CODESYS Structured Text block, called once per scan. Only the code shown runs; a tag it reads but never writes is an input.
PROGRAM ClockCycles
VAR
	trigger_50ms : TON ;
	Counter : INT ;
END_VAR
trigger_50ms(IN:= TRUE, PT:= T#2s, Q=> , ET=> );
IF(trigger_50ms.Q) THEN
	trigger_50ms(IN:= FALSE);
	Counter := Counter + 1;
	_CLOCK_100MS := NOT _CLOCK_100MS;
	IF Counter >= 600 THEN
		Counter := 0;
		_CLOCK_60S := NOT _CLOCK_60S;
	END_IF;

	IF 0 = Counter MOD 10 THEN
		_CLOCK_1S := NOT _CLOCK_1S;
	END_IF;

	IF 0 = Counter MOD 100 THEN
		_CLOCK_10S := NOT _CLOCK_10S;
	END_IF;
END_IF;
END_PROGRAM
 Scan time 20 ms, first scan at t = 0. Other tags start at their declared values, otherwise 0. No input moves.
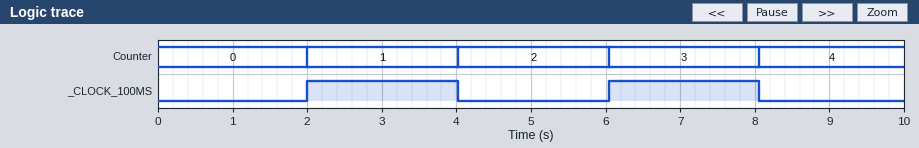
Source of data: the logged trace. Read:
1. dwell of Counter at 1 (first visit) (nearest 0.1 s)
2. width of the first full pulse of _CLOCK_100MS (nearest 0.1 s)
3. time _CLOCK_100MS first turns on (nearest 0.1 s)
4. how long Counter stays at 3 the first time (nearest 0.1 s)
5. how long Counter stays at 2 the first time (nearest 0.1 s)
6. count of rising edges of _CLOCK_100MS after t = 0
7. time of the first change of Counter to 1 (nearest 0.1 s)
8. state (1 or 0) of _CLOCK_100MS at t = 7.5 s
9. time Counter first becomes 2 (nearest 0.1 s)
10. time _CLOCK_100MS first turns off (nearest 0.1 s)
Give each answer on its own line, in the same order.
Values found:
2.0 s
2.0 s
2.0 s
2.0 s
2.0 s
2
2.0 s
1
4.0 s
4.0 s
